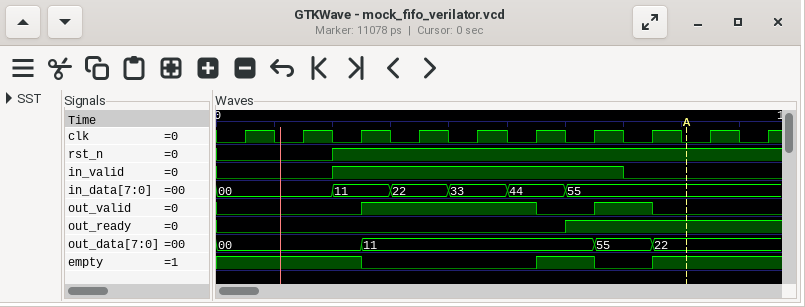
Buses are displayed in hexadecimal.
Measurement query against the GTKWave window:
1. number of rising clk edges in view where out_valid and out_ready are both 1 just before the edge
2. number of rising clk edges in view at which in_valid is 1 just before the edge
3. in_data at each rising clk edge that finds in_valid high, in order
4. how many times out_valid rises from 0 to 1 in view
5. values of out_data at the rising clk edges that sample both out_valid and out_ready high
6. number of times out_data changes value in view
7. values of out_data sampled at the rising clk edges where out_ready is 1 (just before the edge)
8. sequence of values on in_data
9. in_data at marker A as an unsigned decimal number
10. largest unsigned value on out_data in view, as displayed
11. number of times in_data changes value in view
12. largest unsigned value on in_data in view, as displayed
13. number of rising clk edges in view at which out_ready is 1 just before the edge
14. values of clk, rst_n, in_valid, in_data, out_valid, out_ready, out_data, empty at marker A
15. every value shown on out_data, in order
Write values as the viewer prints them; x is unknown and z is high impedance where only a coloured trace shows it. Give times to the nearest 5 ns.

1
5
11, 22, 33, 44, 55
2
55
3
11, 55, 22, 22
00, 11, 22, 33, 44, 55
85
55
5
55
4
clk=0, rst_n=1, in_valid=0, in_data=55, out_valid=0, out_ready=1, out_data=22, empty=1
00, 11, 55, 22
